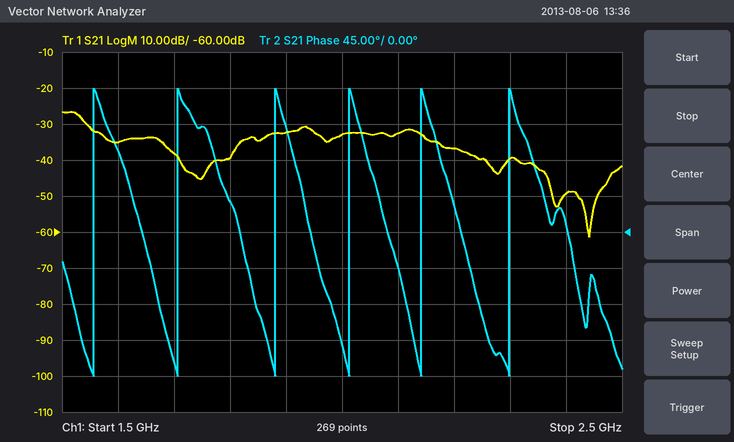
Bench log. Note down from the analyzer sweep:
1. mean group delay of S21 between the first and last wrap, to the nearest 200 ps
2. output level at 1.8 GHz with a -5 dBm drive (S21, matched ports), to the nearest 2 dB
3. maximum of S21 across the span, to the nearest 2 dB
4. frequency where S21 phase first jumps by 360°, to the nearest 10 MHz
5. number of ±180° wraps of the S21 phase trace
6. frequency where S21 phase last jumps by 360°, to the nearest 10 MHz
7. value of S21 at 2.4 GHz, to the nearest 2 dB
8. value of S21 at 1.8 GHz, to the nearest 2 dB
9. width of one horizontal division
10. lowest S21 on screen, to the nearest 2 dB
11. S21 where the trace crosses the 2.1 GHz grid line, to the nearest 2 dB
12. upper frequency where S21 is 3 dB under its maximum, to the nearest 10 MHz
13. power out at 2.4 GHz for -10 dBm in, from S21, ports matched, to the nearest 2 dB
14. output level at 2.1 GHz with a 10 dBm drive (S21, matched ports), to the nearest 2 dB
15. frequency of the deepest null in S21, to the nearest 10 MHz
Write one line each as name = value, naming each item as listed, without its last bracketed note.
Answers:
mean group delay of S21 between the first and last wrap, to the nearest 200 ps = 6.8 ns
output level at 1.8 GHz with a -5 dBm drive (S21, matched ports), to the nearest 2 dB = -44 dBm
maximum of S21 across the span, to the nearest 2 dB = -26 dB
frequency where S21 phase first jumps by 360°, to the nearest 10 MHz = 1.56 GHz
number of ±180° wraps of the S21 phase trace = 6
frequency where S21 phase last jumps by 360°, to the nearest 10 MHz = 2.30 GHz
value of S21 at 2.4 GHz, to the nearest 2 dB = -50 dB
value of S21 at 1.8 GHz, to the nearest 2 dB = -40 dB
width of one horizontal division = 100 MHz
lowest S21 on screen, to the nearest 2 dB = -62 dB
S21 where the trace crosses the 2.1 GHz grid line, to the nearest 2 dB = -32 dB
upper frequency where S21 is 3 dB under its maximum, to the nearest 10 MHz = 1.54 GHz
power out at 2.4 GHz for -10 dBm in, from S21, ports matched, to the nearest 2 dB = -60 dBm
output level at 2.1 GHz with a 10 dBm drive (S21, matched ports), to the nearest 2 dB = -22 dBm
frequency of the deepest null in S21, to the nearest 10 MHz = 2.44 GHz
